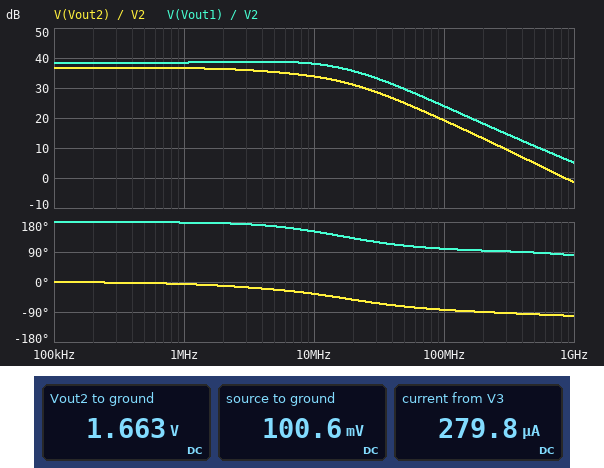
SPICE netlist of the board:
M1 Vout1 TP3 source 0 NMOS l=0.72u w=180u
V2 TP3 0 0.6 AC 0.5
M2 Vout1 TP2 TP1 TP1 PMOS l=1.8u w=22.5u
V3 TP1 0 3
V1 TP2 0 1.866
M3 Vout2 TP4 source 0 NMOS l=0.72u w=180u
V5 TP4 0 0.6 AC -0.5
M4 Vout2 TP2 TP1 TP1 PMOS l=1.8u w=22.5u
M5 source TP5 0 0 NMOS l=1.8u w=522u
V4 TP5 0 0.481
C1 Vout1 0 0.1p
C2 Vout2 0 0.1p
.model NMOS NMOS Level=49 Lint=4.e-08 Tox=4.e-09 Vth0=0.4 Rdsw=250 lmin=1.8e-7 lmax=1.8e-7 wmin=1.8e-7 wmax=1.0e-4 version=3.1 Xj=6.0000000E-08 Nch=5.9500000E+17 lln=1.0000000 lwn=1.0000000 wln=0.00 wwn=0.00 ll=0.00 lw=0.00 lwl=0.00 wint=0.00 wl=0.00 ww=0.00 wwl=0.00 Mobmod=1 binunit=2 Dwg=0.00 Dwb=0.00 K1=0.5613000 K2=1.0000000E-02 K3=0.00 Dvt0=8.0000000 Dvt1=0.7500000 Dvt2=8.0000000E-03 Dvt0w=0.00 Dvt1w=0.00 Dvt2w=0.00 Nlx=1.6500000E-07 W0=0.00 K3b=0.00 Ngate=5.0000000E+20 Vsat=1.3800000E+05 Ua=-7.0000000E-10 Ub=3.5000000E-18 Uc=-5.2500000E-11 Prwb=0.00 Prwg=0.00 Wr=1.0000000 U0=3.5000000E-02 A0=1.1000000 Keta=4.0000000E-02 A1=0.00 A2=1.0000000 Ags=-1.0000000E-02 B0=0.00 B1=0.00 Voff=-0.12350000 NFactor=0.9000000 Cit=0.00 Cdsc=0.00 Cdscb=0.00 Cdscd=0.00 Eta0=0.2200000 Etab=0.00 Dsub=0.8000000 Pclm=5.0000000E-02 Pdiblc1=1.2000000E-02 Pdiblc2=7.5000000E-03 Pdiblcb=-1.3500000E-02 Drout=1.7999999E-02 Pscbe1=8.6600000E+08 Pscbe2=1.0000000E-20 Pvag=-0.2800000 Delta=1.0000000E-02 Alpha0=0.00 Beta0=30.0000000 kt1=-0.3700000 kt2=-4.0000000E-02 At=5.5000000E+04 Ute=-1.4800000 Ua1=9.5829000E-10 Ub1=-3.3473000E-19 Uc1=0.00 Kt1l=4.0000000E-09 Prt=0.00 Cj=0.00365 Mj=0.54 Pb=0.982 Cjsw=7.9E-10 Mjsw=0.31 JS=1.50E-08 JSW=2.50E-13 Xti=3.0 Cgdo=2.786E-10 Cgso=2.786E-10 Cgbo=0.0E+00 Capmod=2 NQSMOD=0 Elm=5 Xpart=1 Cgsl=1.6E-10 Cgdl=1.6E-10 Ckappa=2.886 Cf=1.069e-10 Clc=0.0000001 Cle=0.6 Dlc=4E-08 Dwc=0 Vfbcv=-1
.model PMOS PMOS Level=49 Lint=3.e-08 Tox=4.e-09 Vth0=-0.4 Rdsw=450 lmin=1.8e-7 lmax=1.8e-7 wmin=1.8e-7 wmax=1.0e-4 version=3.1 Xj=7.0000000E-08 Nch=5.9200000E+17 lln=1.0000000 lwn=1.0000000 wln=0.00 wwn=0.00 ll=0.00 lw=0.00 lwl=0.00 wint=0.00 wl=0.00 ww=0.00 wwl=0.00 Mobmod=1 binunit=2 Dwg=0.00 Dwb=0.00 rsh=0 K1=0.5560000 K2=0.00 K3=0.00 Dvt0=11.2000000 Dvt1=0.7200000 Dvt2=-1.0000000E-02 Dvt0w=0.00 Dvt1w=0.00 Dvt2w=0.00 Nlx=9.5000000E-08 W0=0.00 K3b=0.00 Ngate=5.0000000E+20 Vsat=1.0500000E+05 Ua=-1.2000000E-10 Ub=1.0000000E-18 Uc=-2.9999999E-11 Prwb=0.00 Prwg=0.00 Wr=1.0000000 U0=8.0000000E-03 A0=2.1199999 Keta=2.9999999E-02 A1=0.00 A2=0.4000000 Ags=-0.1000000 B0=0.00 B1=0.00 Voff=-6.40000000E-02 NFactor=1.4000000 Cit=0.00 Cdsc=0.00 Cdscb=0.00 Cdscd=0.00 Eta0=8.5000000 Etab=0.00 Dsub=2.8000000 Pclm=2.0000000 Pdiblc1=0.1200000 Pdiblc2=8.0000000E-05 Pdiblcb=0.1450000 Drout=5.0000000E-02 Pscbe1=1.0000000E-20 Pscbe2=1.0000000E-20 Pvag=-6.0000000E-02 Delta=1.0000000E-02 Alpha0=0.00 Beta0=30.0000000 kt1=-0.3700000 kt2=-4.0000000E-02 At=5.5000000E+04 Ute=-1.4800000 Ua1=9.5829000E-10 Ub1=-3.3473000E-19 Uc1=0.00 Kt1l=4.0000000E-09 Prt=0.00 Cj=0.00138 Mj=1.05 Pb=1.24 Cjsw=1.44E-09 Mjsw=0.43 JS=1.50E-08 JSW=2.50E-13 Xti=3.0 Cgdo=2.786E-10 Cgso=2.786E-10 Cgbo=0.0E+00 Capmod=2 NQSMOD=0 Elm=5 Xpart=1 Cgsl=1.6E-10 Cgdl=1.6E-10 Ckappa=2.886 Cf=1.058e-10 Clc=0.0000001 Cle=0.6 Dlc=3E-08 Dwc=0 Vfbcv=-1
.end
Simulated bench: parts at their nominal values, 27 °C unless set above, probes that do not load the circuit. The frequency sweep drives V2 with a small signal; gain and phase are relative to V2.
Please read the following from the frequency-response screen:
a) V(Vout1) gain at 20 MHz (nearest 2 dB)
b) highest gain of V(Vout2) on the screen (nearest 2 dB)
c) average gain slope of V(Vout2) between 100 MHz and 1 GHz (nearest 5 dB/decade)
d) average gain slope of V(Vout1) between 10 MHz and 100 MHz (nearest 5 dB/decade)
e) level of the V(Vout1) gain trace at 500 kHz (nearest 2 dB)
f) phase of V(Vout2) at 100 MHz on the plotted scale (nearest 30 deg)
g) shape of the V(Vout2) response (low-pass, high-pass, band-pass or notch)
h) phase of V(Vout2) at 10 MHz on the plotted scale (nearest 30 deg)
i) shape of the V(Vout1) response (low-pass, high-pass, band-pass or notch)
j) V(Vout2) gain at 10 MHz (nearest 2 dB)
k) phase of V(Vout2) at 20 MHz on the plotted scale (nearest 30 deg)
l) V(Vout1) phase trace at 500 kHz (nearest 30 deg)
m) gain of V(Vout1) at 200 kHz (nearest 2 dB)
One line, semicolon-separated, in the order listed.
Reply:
36 dB; 36 dB; -20 dB/decade; -15 dB/decade; 38 dB; -90 deg; low-pass; -30 deg; low-pass; 34 dB; -60 deg; 180 deg; 38 dB
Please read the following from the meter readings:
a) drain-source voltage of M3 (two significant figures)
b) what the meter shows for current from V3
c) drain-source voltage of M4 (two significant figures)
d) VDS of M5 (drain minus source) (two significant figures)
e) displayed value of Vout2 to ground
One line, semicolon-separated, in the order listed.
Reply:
1.6 V; 279.8 µA; -1.3 V; 100 mV; 1.663 V
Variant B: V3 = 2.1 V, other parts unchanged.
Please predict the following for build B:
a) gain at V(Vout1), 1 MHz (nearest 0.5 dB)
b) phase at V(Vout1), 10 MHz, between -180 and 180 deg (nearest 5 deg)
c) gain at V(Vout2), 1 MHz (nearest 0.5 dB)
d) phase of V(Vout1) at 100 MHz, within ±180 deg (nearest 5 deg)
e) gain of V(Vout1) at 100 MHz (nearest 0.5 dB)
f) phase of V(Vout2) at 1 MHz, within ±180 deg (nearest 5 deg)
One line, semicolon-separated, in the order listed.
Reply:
-60.0 dB; 85 deg; -67.0 dB; 60 deg; -23.0 dB; 90 deg
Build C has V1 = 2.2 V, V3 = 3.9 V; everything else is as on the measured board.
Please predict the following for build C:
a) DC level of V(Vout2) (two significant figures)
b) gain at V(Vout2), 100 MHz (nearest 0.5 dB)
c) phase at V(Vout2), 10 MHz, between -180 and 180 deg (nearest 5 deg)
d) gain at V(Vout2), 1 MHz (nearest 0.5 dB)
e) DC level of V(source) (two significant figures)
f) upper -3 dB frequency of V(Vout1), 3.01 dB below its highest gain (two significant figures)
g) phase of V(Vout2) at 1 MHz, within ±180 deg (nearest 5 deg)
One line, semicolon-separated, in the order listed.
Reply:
3.7 V; 7.5 dB; -5 deg; 9.0 dB; 110 mV; 200 MHz; 0 deg
